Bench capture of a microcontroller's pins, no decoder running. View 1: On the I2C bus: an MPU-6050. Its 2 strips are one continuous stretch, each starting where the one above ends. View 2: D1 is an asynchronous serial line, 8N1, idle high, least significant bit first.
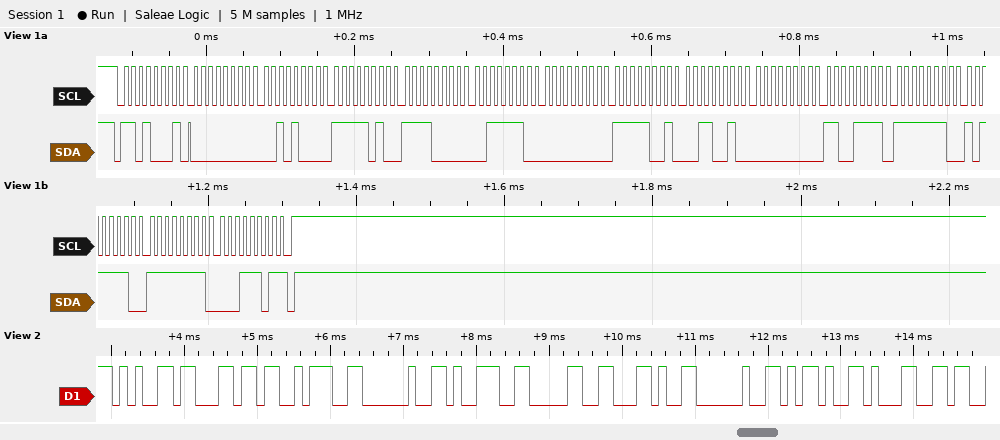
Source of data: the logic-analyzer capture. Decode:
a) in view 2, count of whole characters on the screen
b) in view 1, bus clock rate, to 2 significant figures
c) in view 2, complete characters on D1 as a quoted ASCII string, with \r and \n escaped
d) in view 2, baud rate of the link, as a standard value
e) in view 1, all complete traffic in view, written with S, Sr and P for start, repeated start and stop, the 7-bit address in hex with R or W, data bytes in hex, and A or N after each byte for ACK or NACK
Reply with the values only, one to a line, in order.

10
100 kHz
"el: 90, -1"
9600 baud
S 68R A 00 A 28 A FA A F0 A 3E A 00 A F9 A 32 A 00 A CF A FE A BE A FF A 1D N P
